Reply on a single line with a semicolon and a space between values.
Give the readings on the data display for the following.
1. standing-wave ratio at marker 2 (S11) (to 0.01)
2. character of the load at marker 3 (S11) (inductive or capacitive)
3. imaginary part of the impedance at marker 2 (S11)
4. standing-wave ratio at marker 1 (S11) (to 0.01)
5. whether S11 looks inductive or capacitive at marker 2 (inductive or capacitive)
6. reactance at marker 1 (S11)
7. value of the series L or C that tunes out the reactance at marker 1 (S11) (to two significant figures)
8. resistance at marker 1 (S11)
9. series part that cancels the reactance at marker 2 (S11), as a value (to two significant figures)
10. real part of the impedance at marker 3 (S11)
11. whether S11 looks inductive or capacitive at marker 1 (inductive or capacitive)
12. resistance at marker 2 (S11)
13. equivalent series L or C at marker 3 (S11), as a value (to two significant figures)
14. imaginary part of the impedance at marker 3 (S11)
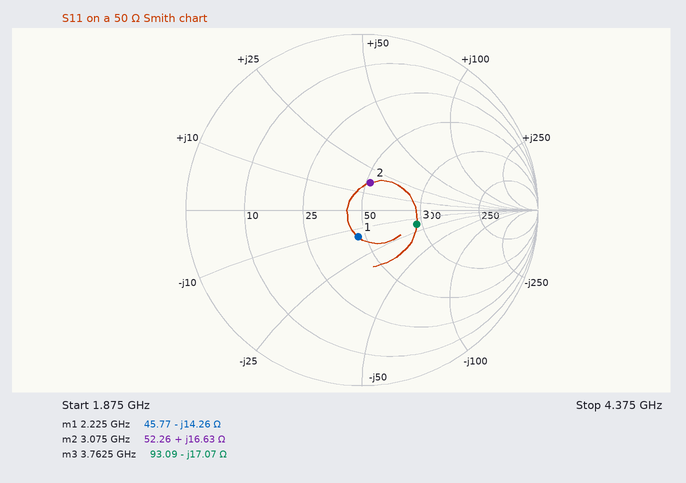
1.39; capacitive; +16.63 Ω; 1.36; inductive; -14.26 Ω; 1.0 nH; 45.77 Ω; 3.1 pF; 93.09 Ω; capacitive; 52.26 Ω; 2.5 pF; -17.07 Ω
